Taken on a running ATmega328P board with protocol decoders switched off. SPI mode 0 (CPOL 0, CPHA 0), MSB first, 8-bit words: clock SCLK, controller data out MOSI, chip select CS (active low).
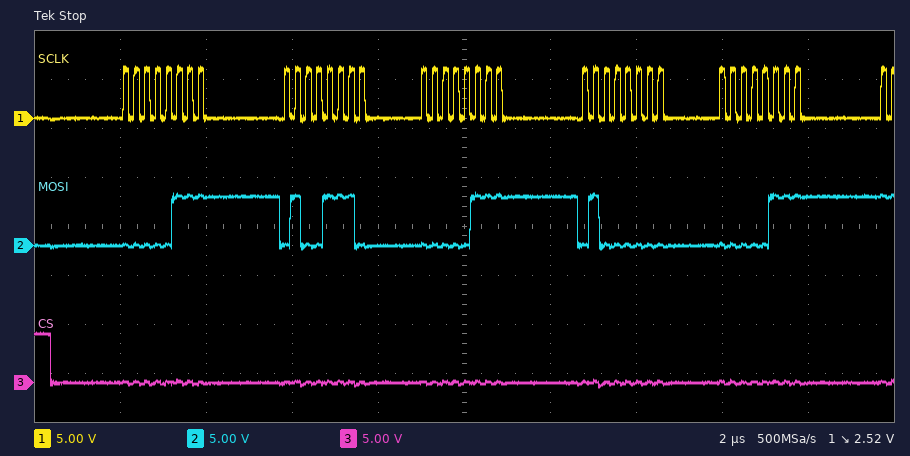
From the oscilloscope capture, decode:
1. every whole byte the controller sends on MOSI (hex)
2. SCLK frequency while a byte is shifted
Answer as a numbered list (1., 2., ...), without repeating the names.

1. 0x07 0x4E 0x07 0x40 0x07
2. 4 MHz
